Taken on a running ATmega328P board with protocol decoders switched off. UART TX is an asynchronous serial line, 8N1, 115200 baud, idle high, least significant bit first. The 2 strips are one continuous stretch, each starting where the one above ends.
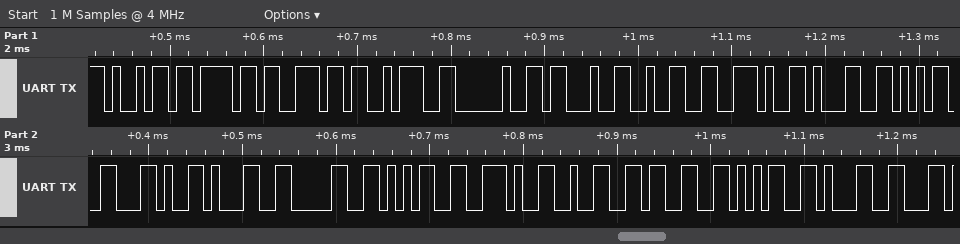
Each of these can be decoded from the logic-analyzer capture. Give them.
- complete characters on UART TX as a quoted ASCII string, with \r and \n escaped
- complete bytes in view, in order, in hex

"ion: #2.15,105.2351"
69 6F 6E 3A 20 23 32 2E 31 35 2C 31 30 35 2E 32 33 35 31
